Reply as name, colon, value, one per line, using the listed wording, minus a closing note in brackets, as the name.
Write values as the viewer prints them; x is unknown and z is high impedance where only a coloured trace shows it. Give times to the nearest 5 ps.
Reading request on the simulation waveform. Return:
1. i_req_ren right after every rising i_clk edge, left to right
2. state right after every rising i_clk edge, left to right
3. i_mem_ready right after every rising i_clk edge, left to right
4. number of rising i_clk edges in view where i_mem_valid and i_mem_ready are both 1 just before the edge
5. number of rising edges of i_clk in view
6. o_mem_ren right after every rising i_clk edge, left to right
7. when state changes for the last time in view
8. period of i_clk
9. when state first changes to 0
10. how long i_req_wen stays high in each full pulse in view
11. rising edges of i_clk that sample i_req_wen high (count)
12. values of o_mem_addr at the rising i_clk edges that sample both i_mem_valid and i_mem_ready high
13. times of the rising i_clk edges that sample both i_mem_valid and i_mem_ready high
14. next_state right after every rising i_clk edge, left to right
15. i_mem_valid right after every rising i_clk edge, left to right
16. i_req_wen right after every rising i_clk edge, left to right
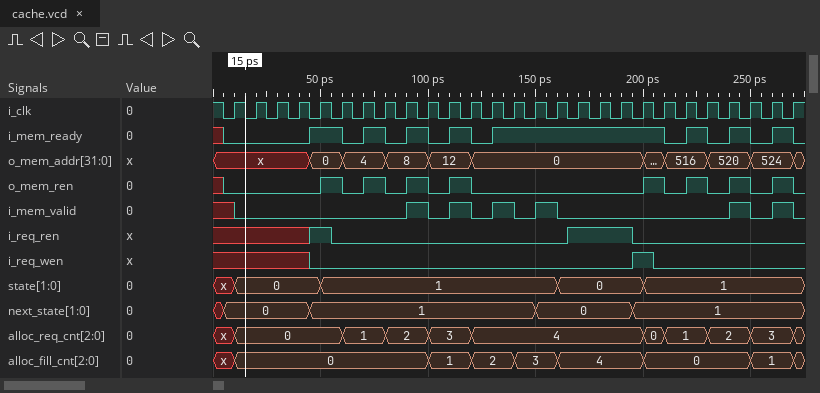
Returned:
i_req_ren right after every rising i_clk edge, left to right: x x x x 1 0 0 0 0 0 0 0 0 0 0 0 1 1 1 0 0 0 0 0 0 0 0
state right after every rising i_clk edge, left to right: 0, 0, 0, 0, 1, 1, 1, 1, 1, 1, 1, 1, 1, 1, 1, 0, 0, 0, 0, 1, 1, 1, 1, 1, 1, 1, 1
i_mem_ready right after every rising i_clk edge, left to right: 0 0 0 0 1 0 1 0 1 0 1 0 1 1 1 1 1 1 1 1 0 1 0 1 0 1 0
number of rising i_clk edges in view where i_mem_valid and i_mem_ready are both 1 just before the edge: 6
number of rising edges of i_clk in view: 27
o_mem_ren right after every rising i_clk edge, left to right: 0 0 0 0 1 0 1 0 1 0 1 0 0 0 0 0 0 0 0 1 0 1 0 1 0 1 0
when state changes for the last time in view: 200 ps
period of i_clk: 10 ps
when state first changes to 0: 10 ps
how long i_req_wen stays high in each full pulse in view: 10 ps
rising edges of i_clk that sample i_req_wen high: 1
values of o_mem_addr at the rising i_clk edges that sample both i_mem_valid and i_mem_ready high: 8, 12, 0, 0, 520, 524
times of the rising i_clk edges that sample both i_mem_valid and i_mem_ready high: 100 ps, 120 ps, 140 ps, 160 ps, 250 ps, 270 ps
next_state right after every rising i_clk edge, left to right: 0, 0, 0, 0, 1, 1, 1, 1, 1, 1, 1, 1, 1, 1, 0, 0, 0, 0, 0, 1, 1, 1, 1, 1, 1, 1, 1
i_mem_valid right after every rising i_clk edge, left to right: 0 0 0 0 0 0 0 0 1 0 1 0 1 0 1 0 0 0 0 0 0 0 0 1 0 1 0
i_req_wen right after every rising i_clk edge, left to right: x x x x 0 0 0 0 0 0 0 0 0 0 0 0 0 0 0 1 0 0 0 0 0 0 0
